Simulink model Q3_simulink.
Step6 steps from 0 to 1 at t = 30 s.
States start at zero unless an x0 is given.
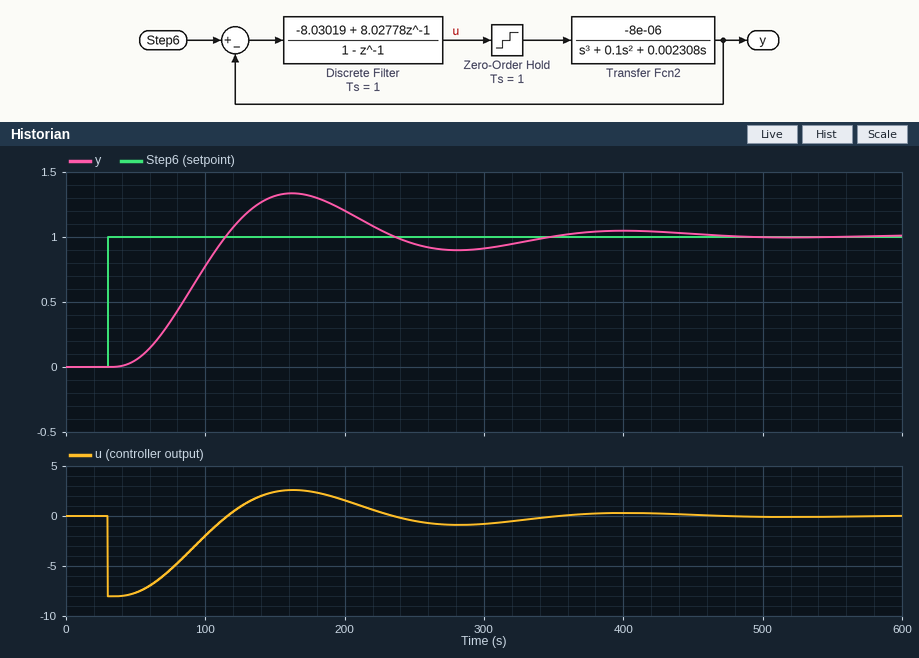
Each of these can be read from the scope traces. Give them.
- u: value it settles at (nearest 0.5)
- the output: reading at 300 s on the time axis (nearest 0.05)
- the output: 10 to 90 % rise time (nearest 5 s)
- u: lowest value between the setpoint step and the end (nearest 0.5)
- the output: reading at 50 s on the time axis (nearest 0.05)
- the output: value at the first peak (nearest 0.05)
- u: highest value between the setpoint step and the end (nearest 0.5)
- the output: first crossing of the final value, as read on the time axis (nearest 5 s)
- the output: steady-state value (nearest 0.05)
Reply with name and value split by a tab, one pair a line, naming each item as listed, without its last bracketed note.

u: value it settles at	0.0
the output: reading at 300 s on the time axis	0.90
the output: 10 to 90 % rise time	50 s
u: lowest value between the setpoint step and the end	-8.0
the output: reading at 50 s on the time axis	0.05
the output: value at the first peak	1.35
u: highest value between the setpoint step and the end	2.5
the output: first crossing of the final value, as read on the time axis	115 s
the output: steady-state value	1.00
